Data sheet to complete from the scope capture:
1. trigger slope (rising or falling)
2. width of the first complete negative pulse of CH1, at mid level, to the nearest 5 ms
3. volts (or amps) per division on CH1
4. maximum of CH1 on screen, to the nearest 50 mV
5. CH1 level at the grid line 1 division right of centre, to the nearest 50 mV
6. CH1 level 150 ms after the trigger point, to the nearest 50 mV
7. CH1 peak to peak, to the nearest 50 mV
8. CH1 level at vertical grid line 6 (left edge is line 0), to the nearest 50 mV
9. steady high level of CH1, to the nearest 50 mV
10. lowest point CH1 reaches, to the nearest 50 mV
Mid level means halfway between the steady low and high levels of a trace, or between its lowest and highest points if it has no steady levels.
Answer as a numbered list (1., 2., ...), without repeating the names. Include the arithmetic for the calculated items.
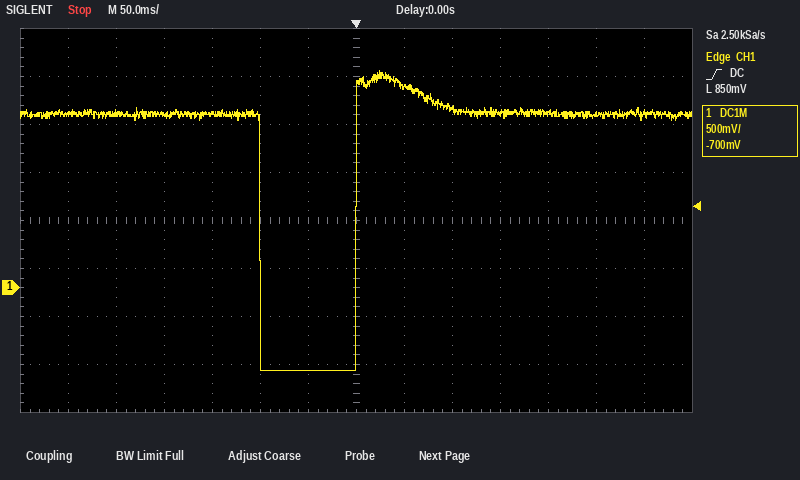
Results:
1. rising
2. 100 ms
3. 500 mV
4. 2.25 V
5. 2.10 V
6. 1.80 V
7. 2.25 V − (-850 mV) = 3.10 V
8. -850 mV
9. 1.80 V
10. -850 mV
